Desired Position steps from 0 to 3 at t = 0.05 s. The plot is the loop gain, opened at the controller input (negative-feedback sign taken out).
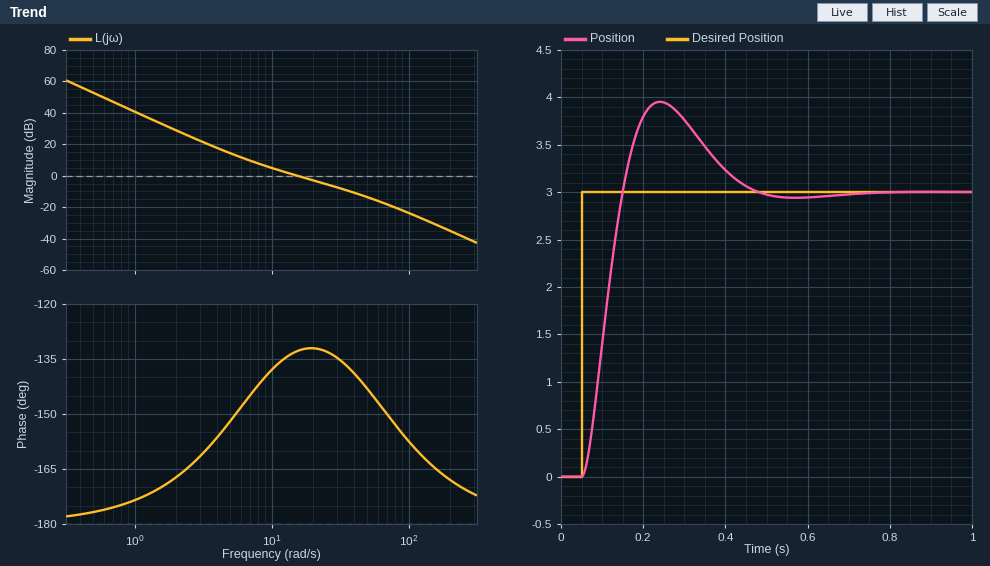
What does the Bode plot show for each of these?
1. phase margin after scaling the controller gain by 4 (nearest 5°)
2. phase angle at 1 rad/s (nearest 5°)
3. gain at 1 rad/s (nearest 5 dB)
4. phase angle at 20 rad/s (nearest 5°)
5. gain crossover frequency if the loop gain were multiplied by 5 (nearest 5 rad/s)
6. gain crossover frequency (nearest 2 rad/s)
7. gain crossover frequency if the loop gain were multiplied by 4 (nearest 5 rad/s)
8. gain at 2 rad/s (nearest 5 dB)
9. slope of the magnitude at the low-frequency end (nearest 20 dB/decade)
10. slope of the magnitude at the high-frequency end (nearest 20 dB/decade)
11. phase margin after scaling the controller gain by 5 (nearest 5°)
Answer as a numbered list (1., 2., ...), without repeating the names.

1. 40°
2. -175°
3. 40 dB
4. -130°
5. 50 rad/s
6. 16 rad/s
7. 45 rad/s
8. 30 dB
9. -40 dB/decade
10. -40 dB/decade
11. 35°
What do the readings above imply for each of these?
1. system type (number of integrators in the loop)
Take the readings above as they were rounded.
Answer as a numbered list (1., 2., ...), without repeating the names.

1. 2
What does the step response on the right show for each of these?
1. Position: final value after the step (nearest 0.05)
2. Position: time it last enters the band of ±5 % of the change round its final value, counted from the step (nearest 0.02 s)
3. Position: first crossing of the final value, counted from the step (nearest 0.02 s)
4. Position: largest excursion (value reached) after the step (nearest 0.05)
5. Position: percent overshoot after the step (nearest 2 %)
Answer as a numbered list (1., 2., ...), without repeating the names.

1. 3.00
2. 0.38 s
3. 0.10 s
4. 3.95
5. 32 %
